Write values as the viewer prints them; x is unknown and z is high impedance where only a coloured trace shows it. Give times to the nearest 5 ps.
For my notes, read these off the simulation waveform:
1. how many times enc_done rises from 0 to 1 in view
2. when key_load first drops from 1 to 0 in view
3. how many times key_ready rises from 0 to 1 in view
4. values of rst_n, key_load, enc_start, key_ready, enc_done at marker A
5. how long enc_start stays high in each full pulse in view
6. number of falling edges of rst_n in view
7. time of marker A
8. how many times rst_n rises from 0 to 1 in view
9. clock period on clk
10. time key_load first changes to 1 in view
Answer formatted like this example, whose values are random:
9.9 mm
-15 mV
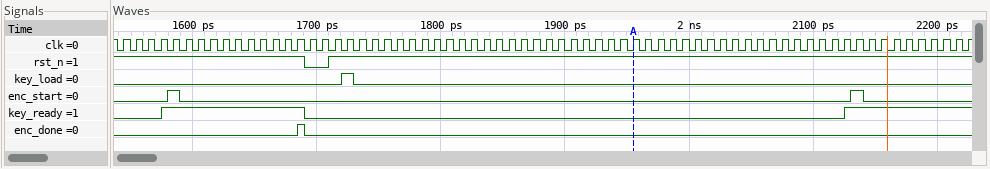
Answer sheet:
1
1730 ps
2
rst_n=1, key_load=0, enc_start=0, key_ready=0, enc_done=0
10 ps, 10 ps
1
1955 ps
1
10 ps
1720 ps
